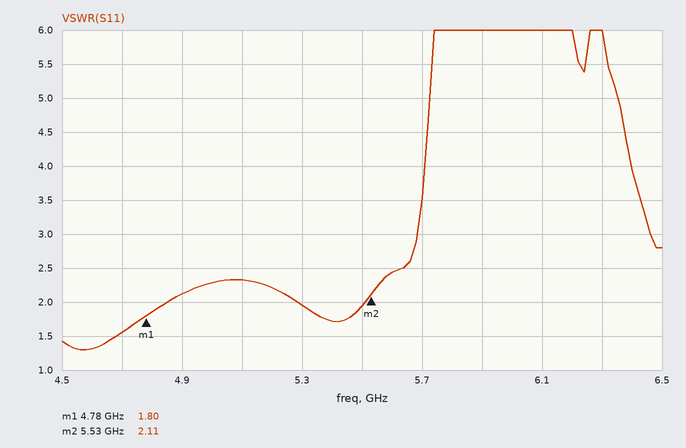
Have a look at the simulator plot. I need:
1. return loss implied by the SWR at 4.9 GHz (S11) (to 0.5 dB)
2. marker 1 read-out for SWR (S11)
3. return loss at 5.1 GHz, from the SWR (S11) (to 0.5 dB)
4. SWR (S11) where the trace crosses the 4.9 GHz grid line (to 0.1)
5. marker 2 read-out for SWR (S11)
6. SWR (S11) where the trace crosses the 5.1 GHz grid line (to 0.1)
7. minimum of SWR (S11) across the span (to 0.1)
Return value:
9.0 dB
1.80
8.0 dB
2.1
2.11
2.3
1.3
